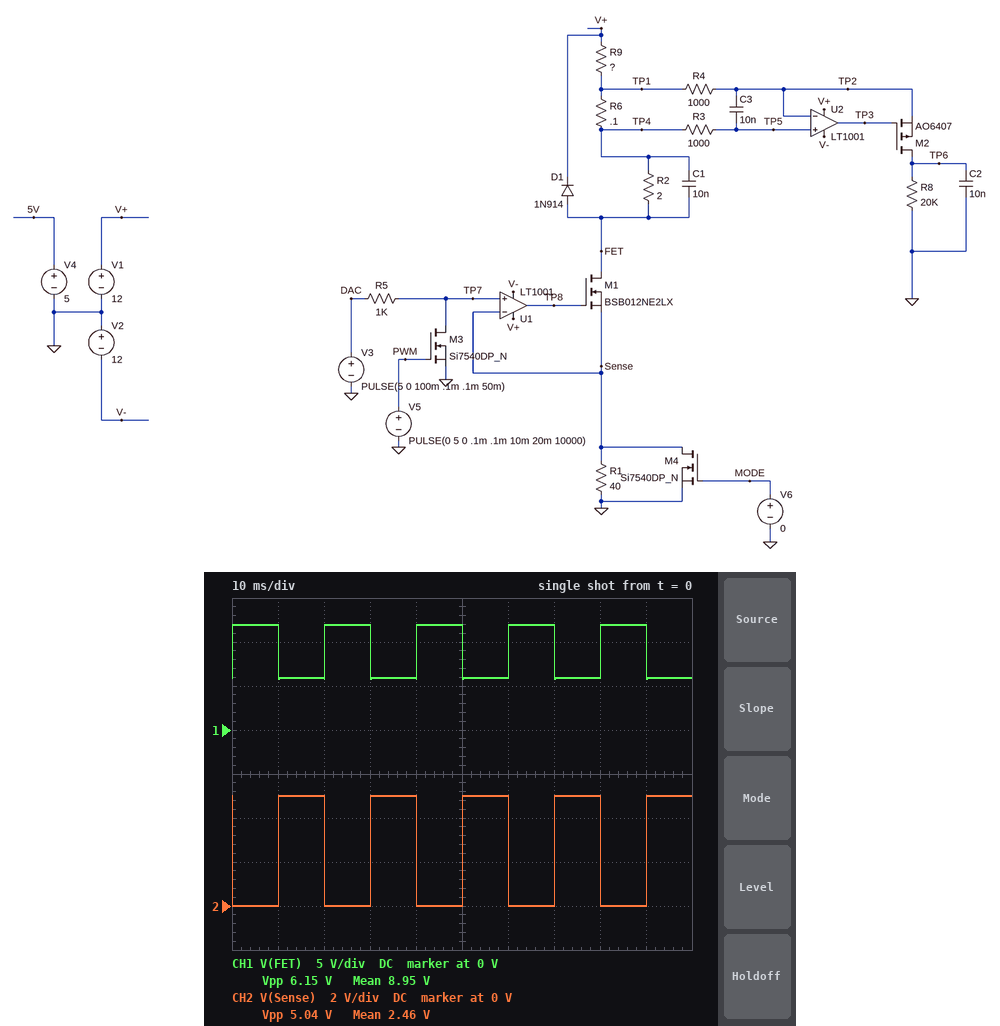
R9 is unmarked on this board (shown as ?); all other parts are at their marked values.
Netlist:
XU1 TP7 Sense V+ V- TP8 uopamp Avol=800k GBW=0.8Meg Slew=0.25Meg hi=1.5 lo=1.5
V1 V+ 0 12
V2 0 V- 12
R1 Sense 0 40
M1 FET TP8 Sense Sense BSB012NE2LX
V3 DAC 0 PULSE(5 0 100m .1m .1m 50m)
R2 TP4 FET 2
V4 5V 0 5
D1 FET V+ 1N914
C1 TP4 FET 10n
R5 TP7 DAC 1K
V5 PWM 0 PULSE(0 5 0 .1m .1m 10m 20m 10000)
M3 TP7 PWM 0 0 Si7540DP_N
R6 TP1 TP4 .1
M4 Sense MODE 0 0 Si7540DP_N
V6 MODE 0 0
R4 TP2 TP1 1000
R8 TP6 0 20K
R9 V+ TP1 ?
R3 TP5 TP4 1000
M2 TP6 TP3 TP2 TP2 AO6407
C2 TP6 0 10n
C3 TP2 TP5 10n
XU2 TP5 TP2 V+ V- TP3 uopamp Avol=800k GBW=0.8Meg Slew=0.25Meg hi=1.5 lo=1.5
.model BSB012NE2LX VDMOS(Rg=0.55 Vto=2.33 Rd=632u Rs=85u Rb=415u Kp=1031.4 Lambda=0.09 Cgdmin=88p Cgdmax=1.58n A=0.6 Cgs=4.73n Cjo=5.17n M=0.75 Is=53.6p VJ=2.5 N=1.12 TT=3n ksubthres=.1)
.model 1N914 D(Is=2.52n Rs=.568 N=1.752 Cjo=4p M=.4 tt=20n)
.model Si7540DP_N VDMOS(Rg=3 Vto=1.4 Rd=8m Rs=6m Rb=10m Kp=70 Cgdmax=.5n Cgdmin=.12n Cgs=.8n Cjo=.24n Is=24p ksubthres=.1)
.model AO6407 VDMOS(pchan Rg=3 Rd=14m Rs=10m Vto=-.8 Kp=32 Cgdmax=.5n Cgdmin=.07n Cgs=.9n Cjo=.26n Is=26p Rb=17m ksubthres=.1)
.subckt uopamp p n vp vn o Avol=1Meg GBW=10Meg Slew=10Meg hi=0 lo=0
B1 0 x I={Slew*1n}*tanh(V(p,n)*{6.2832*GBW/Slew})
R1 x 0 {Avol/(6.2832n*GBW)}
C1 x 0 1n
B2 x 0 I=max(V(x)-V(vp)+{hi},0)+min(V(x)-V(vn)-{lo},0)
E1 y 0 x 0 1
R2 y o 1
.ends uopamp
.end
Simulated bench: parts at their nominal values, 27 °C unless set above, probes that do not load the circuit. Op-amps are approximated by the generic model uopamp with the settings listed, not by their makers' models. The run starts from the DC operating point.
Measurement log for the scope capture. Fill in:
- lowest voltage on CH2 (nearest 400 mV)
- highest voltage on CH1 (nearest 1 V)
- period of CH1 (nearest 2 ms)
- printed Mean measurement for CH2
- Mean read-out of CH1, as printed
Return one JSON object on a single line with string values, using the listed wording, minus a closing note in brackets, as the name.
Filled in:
{"lowest voltage on CH2": "0 V", "highest voltage on CH1": "12 V", "period of CH1": "20 ms", "printed Mean measurement for CH2": "2.46 V", "Mean read-out of CH1, as printed": "8.95 V"}
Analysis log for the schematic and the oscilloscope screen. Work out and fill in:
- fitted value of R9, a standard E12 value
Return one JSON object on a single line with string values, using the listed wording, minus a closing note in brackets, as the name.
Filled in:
{"fitted value of R9, a standard E12 value": "47 Ω"}
